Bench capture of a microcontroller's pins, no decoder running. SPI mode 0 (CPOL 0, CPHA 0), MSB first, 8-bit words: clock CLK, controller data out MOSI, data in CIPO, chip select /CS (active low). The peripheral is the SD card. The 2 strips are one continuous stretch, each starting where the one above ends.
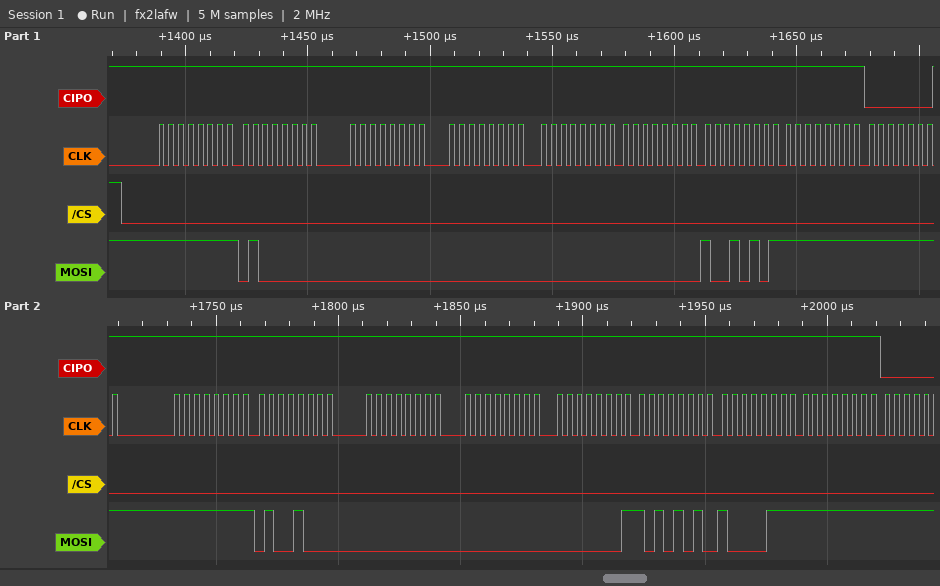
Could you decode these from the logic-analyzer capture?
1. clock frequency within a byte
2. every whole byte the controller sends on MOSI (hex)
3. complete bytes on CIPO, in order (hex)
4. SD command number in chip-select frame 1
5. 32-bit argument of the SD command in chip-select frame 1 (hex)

250 kHz
0xFF 0x40 0x00 0x00 0x00 0x00 0x95 0xFF 0xFF 0xFF 0x48 0x00 0x00 0x01 0xAA 0x87 0xFF
0xFF 0xFF 0xFF 0xFF 0xFF 0xFF 0xFF 0xFF 0x01 0xFF 0xFF 0xFF 0xFF 0xFF 0xFF 0xFF 0xFF
CMD0
0x00000000
